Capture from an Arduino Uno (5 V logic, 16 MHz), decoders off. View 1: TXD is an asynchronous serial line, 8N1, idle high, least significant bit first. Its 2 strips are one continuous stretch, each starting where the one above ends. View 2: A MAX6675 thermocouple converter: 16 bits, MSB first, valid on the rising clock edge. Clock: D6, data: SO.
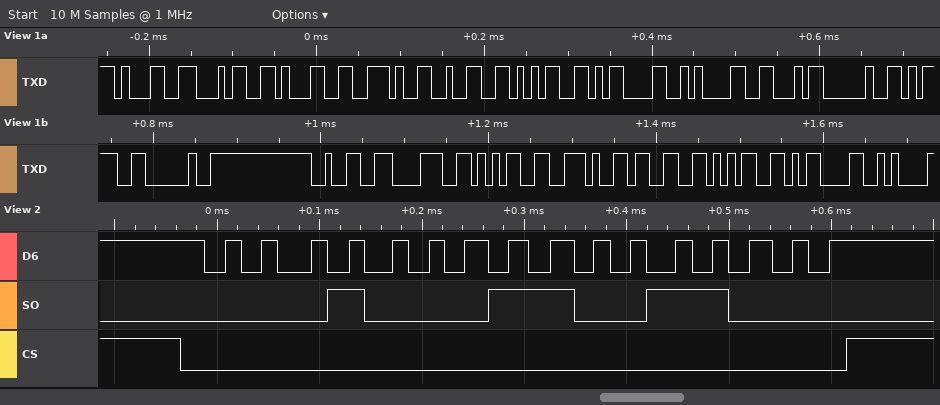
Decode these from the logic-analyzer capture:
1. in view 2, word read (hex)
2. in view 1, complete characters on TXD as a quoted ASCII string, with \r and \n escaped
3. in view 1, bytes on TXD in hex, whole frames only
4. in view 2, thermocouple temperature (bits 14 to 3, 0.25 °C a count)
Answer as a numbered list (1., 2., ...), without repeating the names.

1. 0x1198
2. "141.25\r\nF = 285.35\r\n"
3. 31 34 31 2E 32 35 0D 0A 46 20 3D 20 32 38 35 2E 33 35 0D 0A
4. 140.75 °C
